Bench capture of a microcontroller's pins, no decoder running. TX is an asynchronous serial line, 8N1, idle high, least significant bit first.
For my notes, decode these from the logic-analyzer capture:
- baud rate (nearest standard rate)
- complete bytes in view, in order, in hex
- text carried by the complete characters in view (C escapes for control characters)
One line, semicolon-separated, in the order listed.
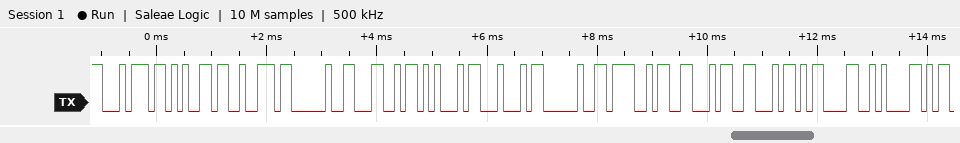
9600 baud; 0x74 0x65 0x72 0x20 0x4C 0x45 0x44 0x20 0x4F 0x46 0x46 0x0D 0x0A; "ter LED OFF\r\n"
